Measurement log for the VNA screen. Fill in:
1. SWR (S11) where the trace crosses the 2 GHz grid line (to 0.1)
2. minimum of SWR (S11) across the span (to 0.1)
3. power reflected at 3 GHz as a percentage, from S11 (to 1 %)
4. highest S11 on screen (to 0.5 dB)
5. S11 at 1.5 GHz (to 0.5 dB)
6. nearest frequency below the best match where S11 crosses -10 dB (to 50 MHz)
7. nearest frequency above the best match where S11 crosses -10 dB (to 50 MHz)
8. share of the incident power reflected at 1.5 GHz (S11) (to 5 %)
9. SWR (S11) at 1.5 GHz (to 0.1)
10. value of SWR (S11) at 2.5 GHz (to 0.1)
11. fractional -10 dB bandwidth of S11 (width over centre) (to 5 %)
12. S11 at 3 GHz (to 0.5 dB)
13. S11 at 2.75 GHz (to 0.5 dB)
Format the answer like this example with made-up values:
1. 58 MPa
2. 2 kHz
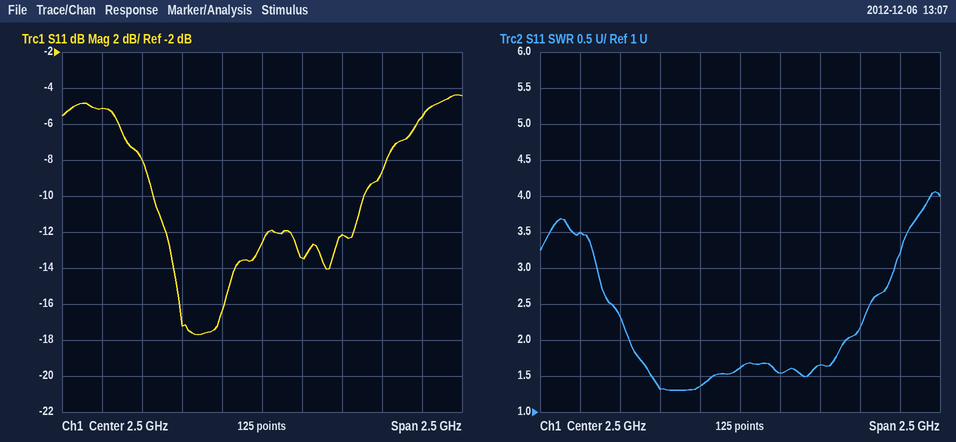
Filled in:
1. 1.3
2. 1.3
3. 6 %
4. -4.5 dB
5. -5.0 dB
6. 1.80 GHz
7. 3.15 GHz
8. 30 %
9. 3.5
10. 1.6
11. 55 %
12. -12.0 dB
13. -13.5 dB
